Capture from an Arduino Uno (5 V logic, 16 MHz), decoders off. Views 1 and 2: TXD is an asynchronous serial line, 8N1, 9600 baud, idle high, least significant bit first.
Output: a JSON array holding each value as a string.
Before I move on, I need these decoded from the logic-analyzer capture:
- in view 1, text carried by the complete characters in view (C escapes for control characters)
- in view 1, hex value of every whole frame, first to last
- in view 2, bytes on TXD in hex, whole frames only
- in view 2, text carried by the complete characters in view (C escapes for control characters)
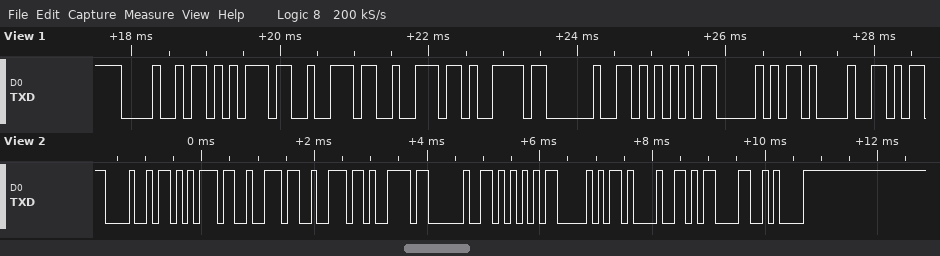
["\"Hurry UP!\"", "48 75 72 72 79 20 55 50 21", "0x48 0x75 0x72 0x72 0x79 0x20 0x55 0x50 0x21 0x0D 0x0A", "\"Hurry UP!\\r\\n\""]
